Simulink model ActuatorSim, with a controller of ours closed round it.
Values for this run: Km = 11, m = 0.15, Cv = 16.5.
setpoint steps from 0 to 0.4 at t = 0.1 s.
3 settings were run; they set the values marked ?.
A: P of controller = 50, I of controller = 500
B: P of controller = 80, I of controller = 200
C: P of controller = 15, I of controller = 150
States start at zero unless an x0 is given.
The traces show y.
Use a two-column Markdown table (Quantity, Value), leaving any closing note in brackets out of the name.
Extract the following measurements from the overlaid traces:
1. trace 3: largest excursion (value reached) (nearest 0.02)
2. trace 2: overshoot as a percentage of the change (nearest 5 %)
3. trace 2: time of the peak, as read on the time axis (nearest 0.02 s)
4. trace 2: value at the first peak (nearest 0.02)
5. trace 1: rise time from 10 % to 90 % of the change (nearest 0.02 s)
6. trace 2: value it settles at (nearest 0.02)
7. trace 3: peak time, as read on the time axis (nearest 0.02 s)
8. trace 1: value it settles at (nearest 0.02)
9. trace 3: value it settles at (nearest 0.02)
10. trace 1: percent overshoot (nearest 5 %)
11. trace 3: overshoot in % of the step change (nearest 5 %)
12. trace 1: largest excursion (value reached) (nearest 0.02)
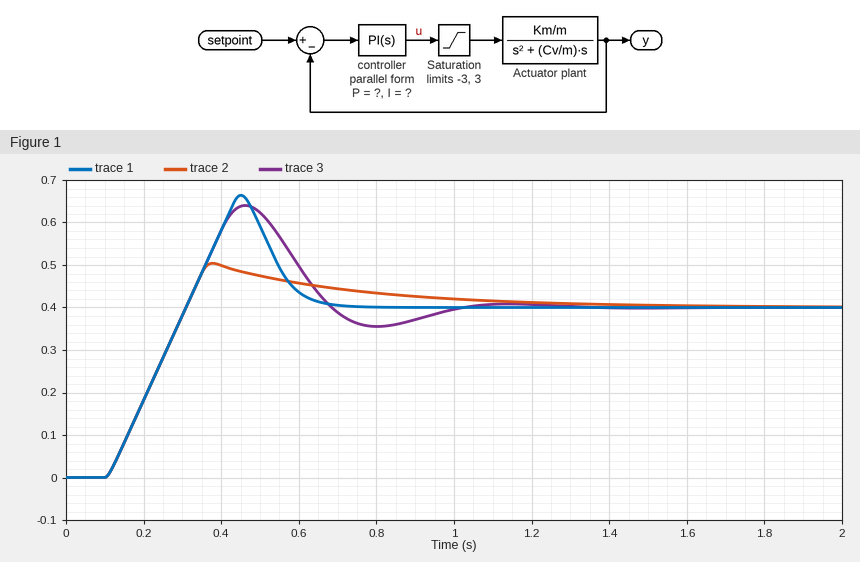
| Quantity | Value |
|---|---|
| trace 3: largest excursion (value reached) | 0.64 |
| trace 2: overshoot as a percentage of the change | 25 % |
| trace 2: time of the peak, as read on the time axis | 0.38 s |
| trace 2: value at the first peak | 0.50 |
| trace 1: rise time from 10 % to 90 % of the change | 0.16 s |
| trace 2: value it settles at | 0.40 |
| trace 3: peak time, as read on the time axis | 0.46 s |
| trace 1: value it settles at | 0.40 |
| trace 3: value it settles at | 0.40 |
| trace 1: percent overshoot | 65 % |
| trace 3: overshoot in % of the step change | 60 % |
| trace 1: largest excursion (value reached) | 0.66 |
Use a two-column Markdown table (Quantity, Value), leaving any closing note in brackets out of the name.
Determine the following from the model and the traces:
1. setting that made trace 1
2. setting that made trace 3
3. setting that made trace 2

| Quantity | Value |
|---|---|
| setting that made trace 1 | A |
| setting that made trace 3 | C |
| setting that made trace 2 | B |
